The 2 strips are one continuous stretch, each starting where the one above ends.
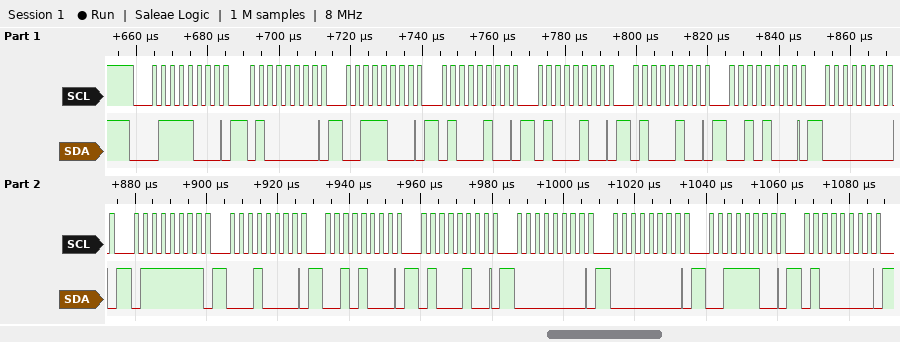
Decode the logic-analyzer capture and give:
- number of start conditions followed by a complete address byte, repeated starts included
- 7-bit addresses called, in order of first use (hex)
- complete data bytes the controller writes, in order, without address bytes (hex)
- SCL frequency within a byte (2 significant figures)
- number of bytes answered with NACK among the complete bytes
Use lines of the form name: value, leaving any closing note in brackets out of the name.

number of start conditions followed by a complete address byte, repeated starts included: 1
7-bit addresses called, in order of first use: 0x3C
complete data bytes the controller writes, in order, without address bytes: 40 38 44 44 44 28 00 7F 10 28 44 00 00 3C 40
SCL frequency within a byte: 400 kHz
number of bytes answered with NACK among the complete bytes: 0
